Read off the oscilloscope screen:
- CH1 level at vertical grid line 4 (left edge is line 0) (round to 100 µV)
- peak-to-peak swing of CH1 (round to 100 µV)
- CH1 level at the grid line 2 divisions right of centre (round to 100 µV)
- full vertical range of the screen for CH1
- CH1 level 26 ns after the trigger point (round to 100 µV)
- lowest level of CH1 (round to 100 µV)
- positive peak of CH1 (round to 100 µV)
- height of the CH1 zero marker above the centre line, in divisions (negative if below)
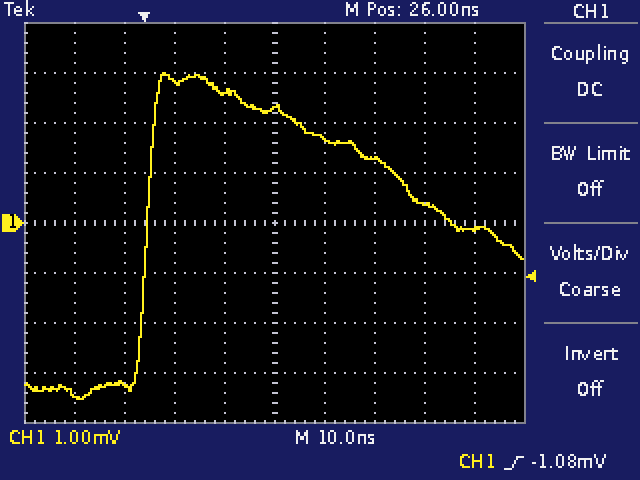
2.6 mV
6.5 mV
1.3 mV
8 mV
2.3 mV
-3.5 mV
3.0 mV
0.0 div
